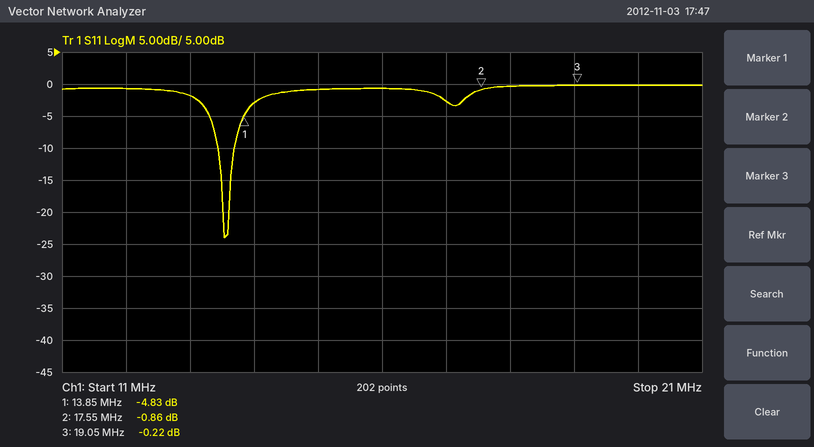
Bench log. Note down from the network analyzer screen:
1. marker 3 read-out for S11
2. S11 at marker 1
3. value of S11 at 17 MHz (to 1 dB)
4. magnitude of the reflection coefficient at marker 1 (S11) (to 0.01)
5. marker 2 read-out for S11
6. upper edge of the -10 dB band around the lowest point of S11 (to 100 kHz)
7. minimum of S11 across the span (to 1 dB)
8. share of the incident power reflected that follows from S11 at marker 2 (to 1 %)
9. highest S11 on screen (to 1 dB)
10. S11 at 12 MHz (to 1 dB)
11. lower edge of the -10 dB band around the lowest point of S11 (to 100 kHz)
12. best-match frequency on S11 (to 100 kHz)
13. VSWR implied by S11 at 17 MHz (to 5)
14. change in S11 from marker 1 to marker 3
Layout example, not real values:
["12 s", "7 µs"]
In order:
["-0.22 dB", "-4.83 dB", "-3 dB", "0.57", "-0.86 dB", "13.7 MHz", "-24 dB", "82 %", "0 dB", "-1 dB", "13.4 MHz", "13.5 MHz", "5", "4.61 dB"]
